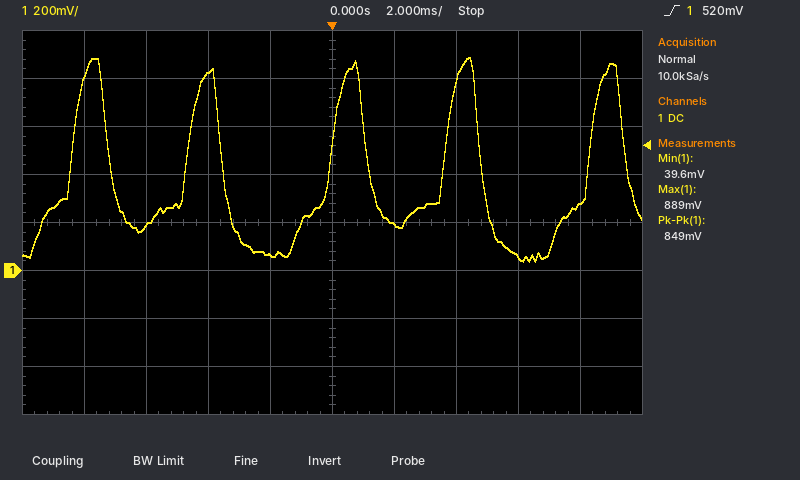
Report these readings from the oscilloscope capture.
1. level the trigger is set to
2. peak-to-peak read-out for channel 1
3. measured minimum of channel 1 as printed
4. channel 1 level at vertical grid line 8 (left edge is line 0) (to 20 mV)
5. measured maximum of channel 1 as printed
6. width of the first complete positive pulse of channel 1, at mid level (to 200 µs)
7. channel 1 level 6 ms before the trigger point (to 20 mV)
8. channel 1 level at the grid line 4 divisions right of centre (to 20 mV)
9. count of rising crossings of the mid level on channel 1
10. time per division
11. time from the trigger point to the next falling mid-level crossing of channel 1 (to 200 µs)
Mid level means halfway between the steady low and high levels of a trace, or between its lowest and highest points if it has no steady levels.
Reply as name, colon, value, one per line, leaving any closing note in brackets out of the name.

level the trigger is set to: 520 mV
peak-to-peak read-out for channel 1: 849 mV
measured minimum of channel 1 as printed: 39.6 mV
channel 1 level at vertical grid line 8 (left edge is line 0): 60 mV
measured maximum of channel 1 as printed: 889 mV
width of the first complete positive pulse of channel 1, at mid level: 1.2 ms
channel 1 level 6 ms before the trigger point: 180 mV
channel 1 level at the grid line 4 divisions right of centre: 280 mV
count of rising crossings of the mid level on channel 1: 5
time per division: 2 ms
time from the trigger point to the next falling mid-level crossing of channel 1: 1.2 ms
